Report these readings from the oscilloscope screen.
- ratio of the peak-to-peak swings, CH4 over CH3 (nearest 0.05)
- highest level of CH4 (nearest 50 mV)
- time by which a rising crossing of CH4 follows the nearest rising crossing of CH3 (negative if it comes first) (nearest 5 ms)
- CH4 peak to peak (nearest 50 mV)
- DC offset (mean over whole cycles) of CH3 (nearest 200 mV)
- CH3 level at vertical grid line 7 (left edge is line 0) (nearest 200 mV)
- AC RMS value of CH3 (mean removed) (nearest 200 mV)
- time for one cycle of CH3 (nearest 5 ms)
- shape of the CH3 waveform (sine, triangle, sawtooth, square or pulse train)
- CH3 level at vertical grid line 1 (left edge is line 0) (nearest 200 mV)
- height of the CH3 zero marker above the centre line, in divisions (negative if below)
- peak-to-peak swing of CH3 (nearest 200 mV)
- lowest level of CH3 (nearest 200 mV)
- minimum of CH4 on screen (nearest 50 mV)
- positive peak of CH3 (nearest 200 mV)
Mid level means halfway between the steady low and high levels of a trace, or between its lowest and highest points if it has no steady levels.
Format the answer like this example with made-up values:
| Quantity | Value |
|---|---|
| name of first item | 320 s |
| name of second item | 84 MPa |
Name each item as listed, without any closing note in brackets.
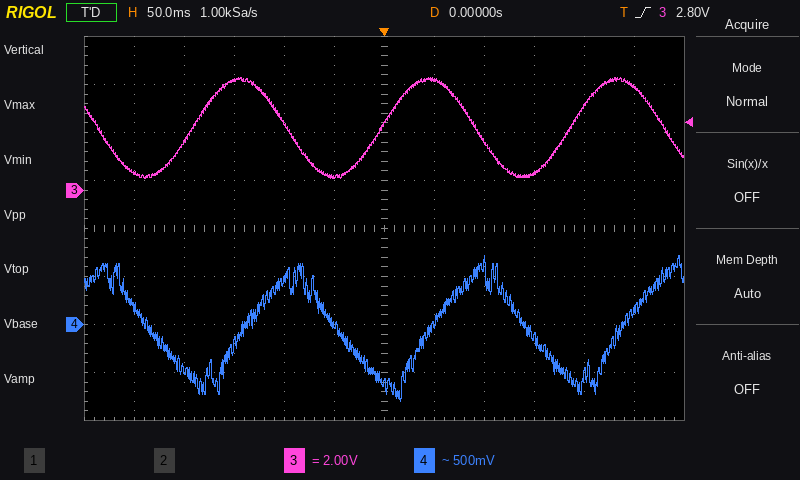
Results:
| Quantity | Value |
|---|---|
| ratio of the peak-to-peak swings, CH4 over CH3 | 0.35 |
| highest level of CH4 | 700 mV |
| time by which a rising crossing of CH4 follows the nearest rising crossing of CH3 (negative if it comes first) | +50 ms |
| CH4 peak to peak | 1.50 V |
| DC offset (mean over whole cycles) of CH3 | 2.6 V |
| CH3 level at vertical grid line 7 (left edge is line 0) | 4.6 V |
| AC RMS value of CH3 (mean removed) | 1.4 V |
| time for one cycle of CH3 | 190 ms |
| shape of the CH3 waveform | sine |
| CH3 level at vertical grid line 1 (left edge is line 0) | 800 mV |
| height of the CH3 zero marker above the centre line, in divisions | +0.8 div |
| peak-to-peak swing of CH3 | 4.2 V |
| lowest level of CH3 | 400 mV |
| minimum of CH4 on screen | -800 mV |
| positive peak of CH3 | 4.6 V |
